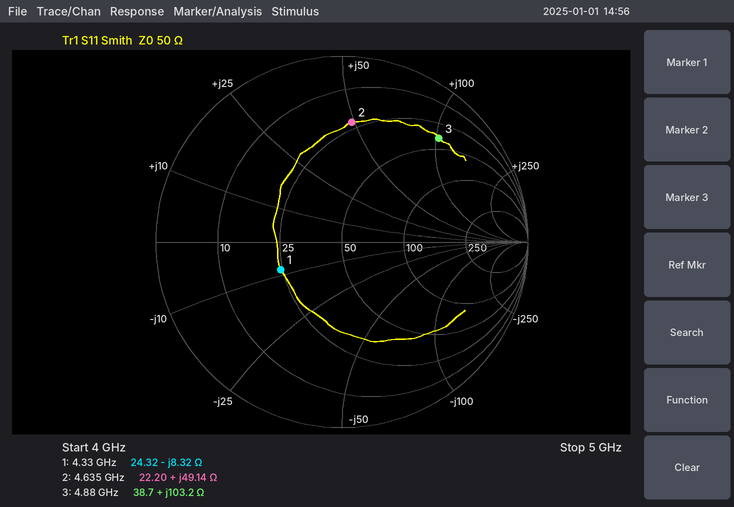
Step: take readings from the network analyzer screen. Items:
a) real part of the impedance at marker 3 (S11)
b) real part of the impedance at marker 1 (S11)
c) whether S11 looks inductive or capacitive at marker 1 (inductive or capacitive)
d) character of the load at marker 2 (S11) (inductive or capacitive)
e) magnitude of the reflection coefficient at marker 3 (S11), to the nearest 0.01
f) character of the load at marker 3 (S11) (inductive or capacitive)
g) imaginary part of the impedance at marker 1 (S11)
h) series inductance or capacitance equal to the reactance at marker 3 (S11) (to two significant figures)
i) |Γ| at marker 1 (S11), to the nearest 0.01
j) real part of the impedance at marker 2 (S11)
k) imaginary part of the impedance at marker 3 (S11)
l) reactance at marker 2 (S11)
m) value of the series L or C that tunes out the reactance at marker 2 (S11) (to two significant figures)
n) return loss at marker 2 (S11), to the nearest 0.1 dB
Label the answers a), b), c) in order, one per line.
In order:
a) 38.7 Ω
b) 24.32 Ω
c) capacitive
d) inductive
e) 0.76
f) inductive
g) -8.32 Ω
h) 3.4 nH
i) 0.36
j) 22.20 Ω
k) +103.2 Ω
l) +49.14 Ω
m) 700 fF
n) 3.8 dB
